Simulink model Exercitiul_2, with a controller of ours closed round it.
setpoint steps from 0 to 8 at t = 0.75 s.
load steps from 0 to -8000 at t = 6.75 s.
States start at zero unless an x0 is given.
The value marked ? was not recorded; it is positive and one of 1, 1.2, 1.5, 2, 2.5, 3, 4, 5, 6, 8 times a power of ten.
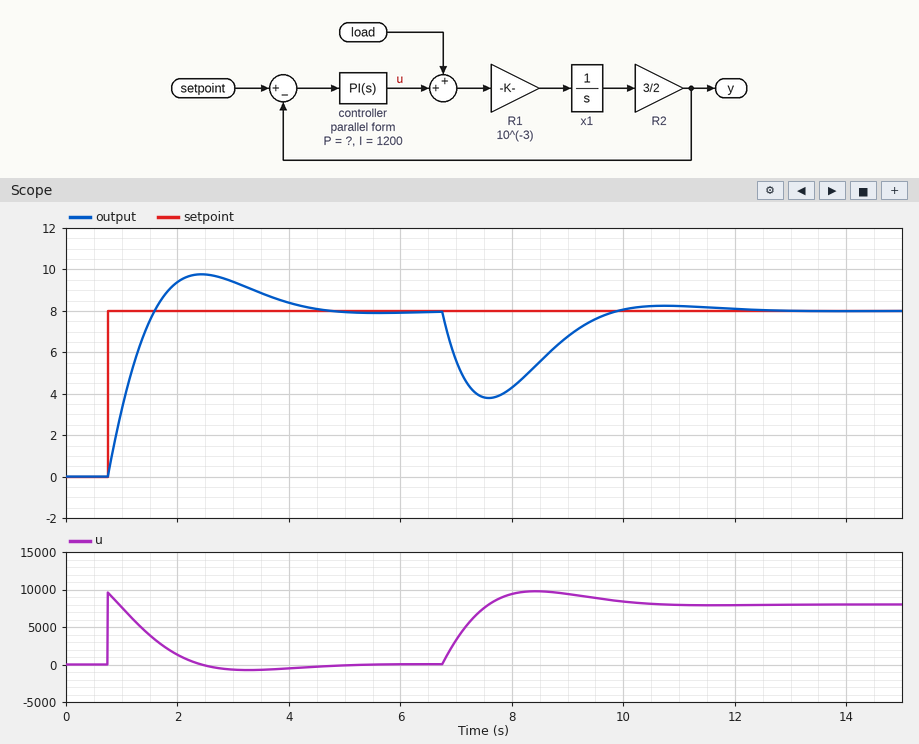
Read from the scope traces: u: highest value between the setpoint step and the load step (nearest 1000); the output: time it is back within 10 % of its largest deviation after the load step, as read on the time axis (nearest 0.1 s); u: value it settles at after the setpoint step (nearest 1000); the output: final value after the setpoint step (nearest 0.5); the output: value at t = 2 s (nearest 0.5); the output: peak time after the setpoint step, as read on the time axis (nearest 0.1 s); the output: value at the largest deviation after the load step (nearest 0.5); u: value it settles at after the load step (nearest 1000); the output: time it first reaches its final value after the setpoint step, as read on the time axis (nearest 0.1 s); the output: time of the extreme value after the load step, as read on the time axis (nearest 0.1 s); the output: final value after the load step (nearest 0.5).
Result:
10000
9.5 s
0
8.0
9.5
2.4 s
4.0
8000
1.6 s
7.6 s
8.0
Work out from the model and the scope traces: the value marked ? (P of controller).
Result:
1200
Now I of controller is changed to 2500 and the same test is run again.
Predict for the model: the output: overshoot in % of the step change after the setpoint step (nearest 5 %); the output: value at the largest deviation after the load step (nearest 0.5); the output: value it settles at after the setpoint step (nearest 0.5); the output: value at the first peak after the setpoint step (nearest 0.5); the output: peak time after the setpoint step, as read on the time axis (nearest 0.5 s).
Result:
30 %
4.5
8.0
10.5
2.0 s
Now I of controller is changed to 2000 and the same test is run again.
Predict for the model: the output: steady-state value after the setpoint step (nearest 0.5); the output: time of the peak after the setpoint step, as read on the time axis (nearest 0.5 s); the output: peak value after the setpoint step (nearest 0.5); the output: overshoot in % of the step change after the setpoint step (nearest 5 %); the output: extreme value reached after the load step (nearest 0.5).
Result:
8.0
2.0 s
10.5
30 %
4.5
